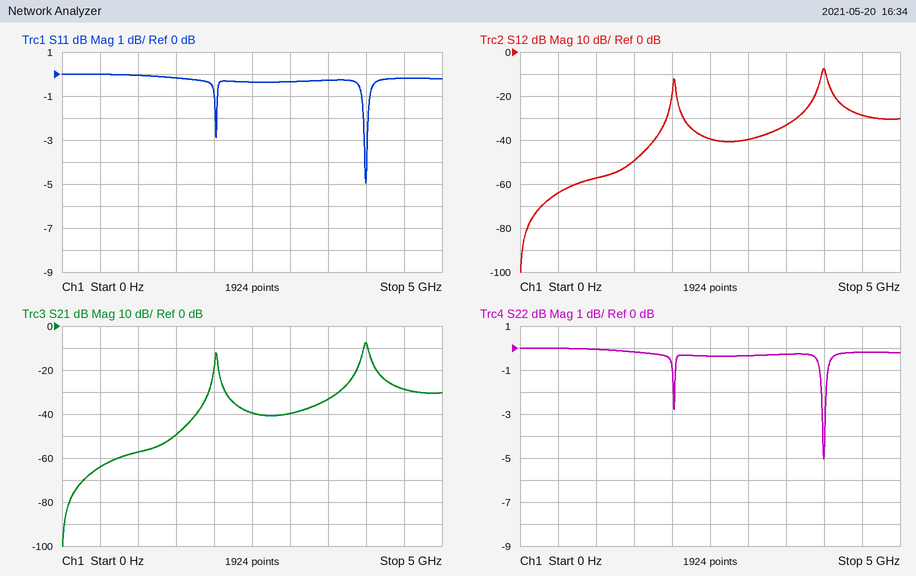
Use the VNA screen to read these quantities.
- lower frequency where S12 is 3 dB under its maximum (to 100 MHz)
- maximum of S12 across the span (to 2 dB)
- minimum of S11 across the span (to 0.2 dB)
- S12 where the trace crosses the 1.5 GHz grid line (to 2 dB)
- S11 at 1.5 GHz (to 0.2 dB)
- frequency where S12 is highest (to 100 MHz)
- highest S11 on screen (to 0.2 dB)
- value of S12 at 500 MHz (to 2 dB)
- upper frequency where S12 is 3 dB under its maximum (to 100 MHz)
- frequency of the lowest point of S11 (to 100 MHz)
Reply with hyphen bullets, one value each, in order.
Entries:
- 4.0 GHz
- -8 dB
- -5.0 dB
- -50 dB
- -0.2 dB
- 4.0 GHz
- 0.0 dB
- -64 dB
- 4.0 GHz
- 4.0 GHz
